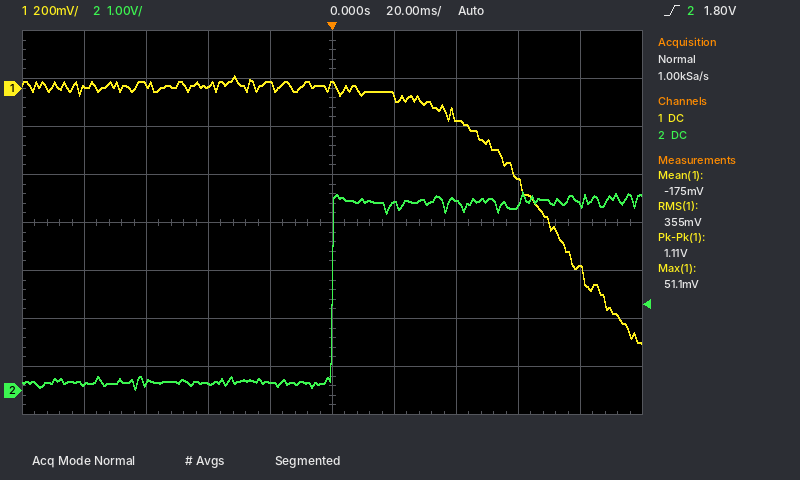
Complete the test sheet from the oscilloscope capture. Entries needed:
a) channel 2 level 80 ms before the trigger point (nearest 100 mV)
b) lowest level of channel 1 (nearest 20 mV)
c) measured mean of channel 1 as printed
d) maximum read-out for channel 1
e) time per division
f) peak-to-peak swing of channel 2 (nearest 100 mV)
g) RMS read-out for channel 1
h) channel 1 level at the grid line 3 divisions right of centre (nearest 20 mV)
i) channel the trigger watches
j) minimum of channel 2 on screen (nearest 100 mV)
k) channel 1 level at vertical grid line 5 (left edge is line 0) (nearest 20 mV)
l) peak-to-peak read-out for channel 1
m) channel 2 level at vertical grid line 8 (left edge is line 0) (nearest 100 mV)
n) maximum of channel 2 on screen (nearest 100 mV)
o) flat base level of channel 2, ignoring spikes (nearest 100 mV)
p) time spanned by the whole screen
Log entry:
100 mV
-1.06 V
-175 mV
51.1 mV
20 ms
4.1 V
355 mV
-380 mV
channel 2
0.0 V
20 mV
1.11 V
3.9 V
4.1 V
200 mV
200 ms
